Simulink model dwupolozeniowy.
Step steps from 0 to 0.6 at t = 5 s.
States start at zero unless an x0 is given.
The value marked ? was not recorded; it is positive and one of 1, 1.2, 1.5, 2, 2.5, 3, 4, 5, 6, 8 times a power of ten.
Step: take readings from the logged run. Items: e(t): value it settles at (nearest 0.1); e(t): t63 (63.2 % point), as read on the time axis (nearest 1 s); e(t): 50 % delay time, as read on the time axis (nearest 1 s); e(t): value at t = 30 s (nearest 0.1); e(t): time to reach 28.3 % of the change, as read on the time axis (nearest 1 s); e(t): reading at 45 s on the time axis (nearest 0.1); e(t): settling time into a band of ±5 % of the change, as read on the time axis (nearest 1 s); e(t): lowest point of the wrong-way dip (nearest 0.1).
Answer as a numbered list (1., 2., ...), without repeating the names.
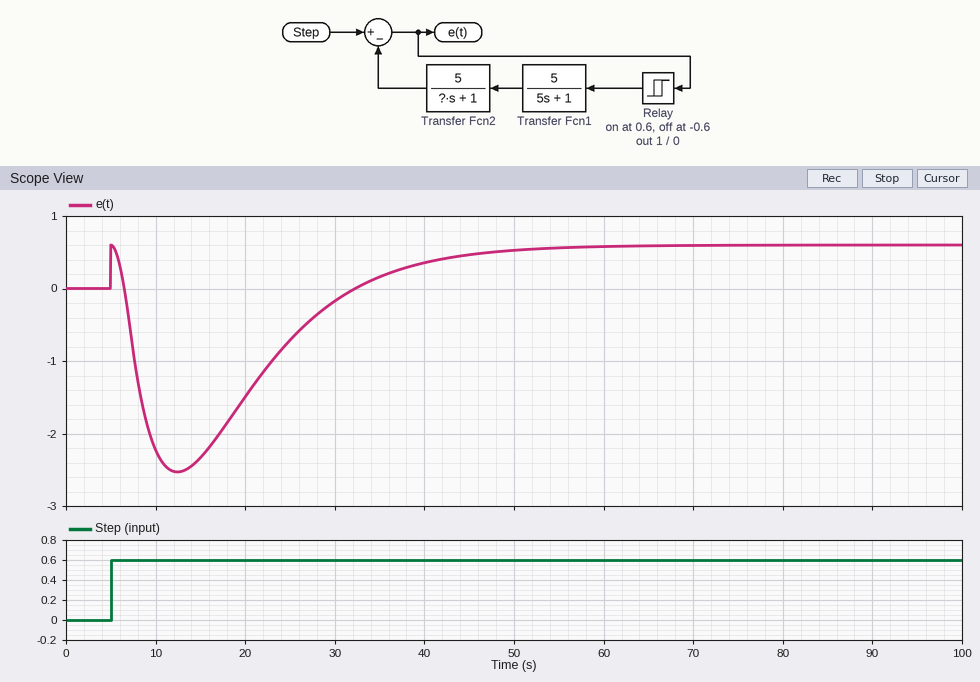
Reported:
1. 0.6
2. 5 s
3. 5 s
4. -0.2
5. 5 s
6. 0.5
7. 57 s
8. -2.5
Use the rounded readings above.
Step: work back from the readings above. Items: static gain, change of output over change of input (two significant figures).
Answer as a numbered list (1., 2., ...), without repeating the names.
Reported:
1. 1.0
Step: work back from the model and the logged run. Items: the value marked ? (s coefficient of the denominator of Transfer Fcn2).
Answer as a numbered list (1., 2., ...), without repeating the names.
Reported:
1. 8
